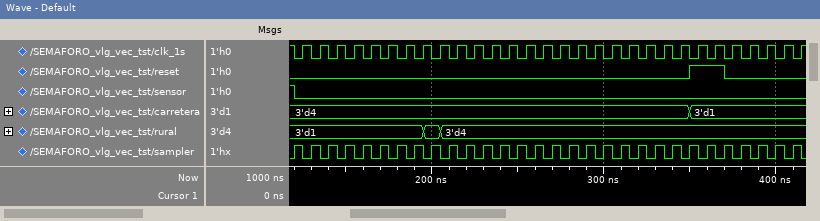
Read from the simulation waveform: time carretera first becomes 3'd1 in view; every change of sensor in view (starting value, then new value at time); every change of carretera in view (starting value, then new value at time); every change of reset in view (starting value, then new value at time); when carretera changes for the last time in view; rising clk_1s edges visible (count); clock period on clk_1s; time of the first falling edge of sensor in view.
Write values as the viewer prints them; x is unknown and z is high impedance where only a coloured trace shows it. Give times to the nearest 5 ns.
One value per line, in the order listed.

350 ns
1, 0 at 120 ns
3'd4, 3'd1 at 350 ns
0, 1 at 350 ns, 0 at 370 ns
350 ns
30
10 ns
120 ns
